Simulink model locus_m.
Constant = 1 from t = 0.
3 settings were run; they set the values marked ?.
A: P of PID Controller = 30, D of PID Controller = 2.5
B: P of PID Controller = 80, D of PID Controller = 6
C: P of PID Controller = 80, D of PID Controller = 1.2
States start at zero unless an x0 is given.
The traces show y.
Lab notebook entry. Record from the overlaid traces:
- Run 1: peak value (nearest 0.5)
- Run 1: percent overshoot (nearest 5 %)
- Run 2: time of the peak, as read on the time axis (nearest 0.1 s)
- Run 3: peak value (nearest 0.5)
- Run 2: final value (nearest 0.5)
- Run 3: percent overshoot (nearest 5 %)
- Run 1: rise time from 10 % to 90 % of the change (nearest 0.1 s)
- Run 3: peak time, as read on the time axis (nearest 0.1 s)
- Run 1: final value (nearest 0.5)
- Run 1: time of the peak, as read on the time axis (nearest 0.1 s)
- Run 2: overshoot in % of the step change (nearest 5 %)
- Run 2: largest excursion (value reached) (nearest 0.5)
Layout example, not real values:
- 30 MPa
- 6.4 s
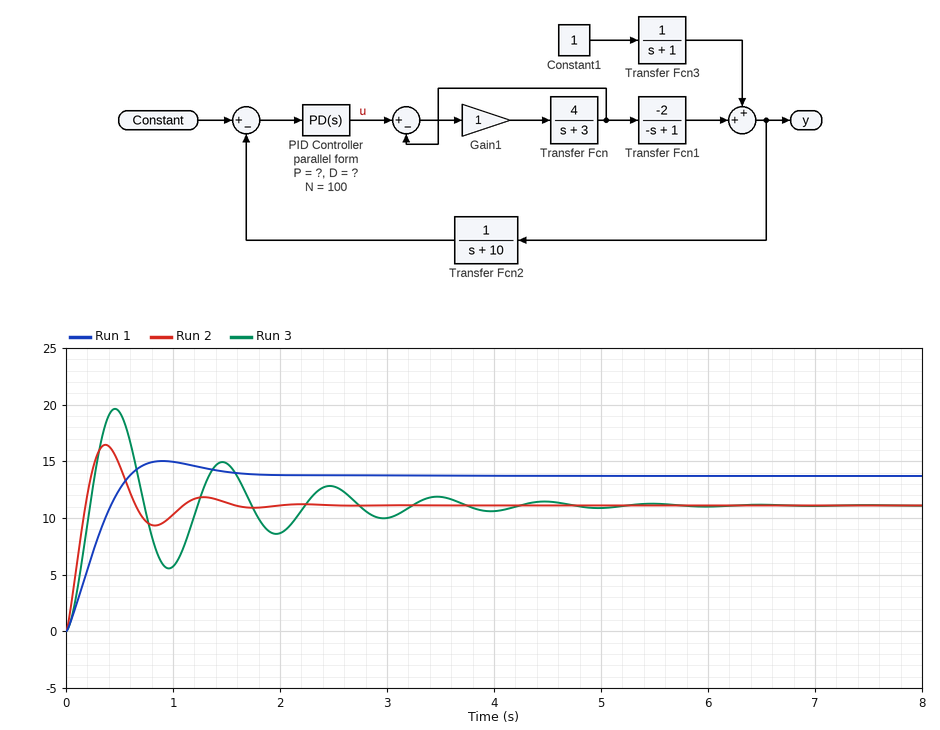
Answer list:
- 15.0
- 10 %
- 0.4 s
- 19.5
- 11.0
- 75 %
- 0.4 s
- 0.5 s
- 13.5
- 0.9 s
- 50 %
- 16.5
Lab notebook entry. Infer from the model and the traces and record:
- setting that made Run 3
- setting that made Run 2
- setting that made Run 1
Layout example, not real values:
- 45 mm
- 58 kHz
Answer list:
- C
- B
- A
